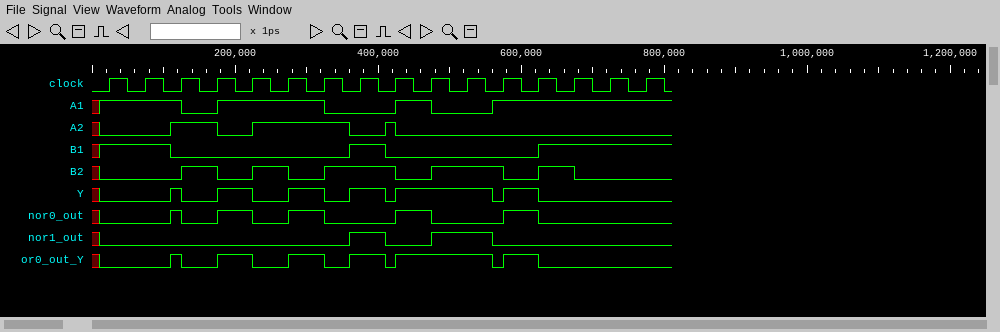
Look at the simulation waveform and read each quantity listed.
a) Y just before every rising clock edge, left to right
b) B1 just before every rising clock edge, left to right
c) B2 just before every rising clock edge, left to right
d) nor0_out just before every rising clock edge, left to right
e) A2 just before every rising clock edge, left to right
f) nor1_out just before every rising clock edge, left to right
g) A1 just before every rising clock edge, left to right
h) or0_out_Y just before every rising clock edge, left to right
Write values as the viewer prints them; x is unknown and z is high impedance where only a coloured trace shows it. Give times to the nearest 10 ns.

0 0 1 0 1 0 1 1 0 1 1 0 1 0 0 0
1 1 0 0 0 0 0 1 0 0 0 0 0 1 1 1
0 0 0 1 0 1 0 1 1 0 1 1 0 1 0 0
0 0 1 0 1 0 1 0 0 1 0 0 1 0 0 0
0 0 1 1 0 1 1 0 1 0 0 0 0 0 0 0
0 0 0 0 0 0 0 1 0 0 1 0 0 0 0 0
1 1 1 0 1 1 1 0 0 1 0 1 1 1 1 1
0 0 1 0 1 0 1 1 0 1 1 0 1 0 0 0
